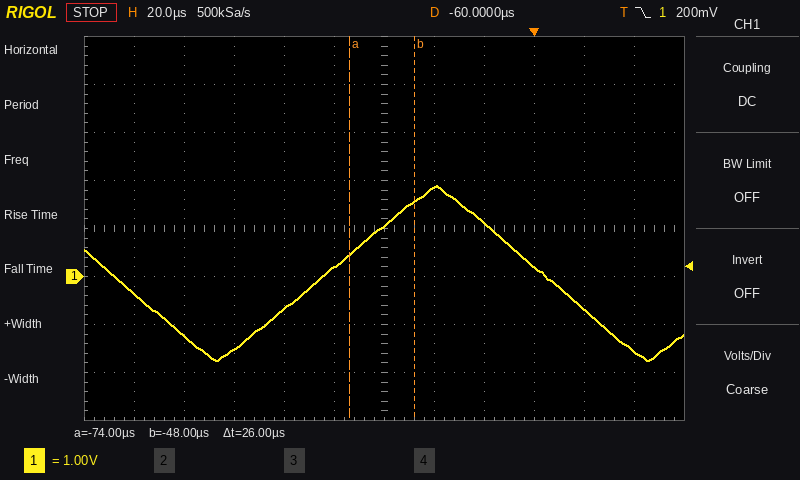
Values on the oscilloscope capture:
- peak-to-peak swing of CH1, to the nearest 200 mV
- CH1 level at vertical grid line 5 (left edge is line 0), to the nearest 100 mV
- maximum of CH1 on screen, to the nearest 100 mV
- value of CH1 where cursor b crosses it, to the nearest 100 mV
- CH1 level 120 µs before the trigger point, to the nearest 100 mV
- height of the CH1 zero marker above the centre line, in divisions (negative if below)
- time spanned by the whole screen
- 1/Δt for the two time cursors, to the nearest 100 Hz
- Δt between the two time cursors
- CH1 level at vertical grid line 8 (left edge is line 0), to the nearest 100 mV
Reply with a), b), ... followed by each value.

a) 3.6 V
b) 200 mV
c) 1.9 V
d) 1.6 V
e) -1.5 V
f) -1.0 div
g) 240 µs
h) 38.5 kHz
i) 26 µs
j) 1.1 V
